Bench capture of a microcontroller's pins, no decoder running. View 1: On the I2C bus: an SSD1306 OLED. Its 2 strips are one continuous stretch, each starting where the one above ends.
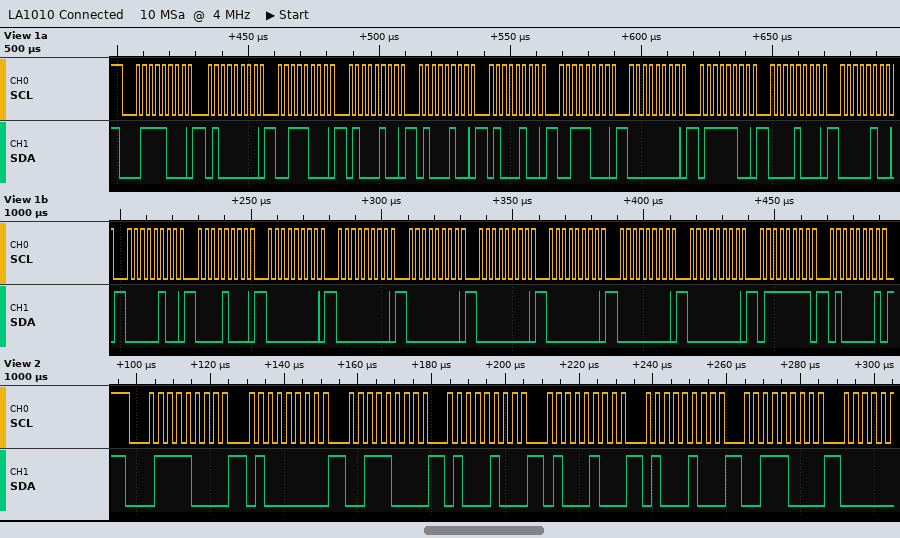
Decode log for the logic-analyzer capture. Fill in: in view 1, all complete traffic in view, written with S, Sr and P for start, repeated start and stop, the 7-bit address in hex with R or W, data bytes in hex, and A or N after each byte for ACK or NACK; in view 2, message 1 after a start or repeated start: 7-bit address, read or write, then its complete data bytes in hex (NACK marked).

S 3CW A 40 A 38 A 44 A 44 A 44 A 38 A 00 A 7C A 08 A 04 A 04 A 08 A 00 A 00 A 00 A 00 A 00 A 00 A 00 A 7F A 41 A
0x3C write: 40 38 44 44 44 38
